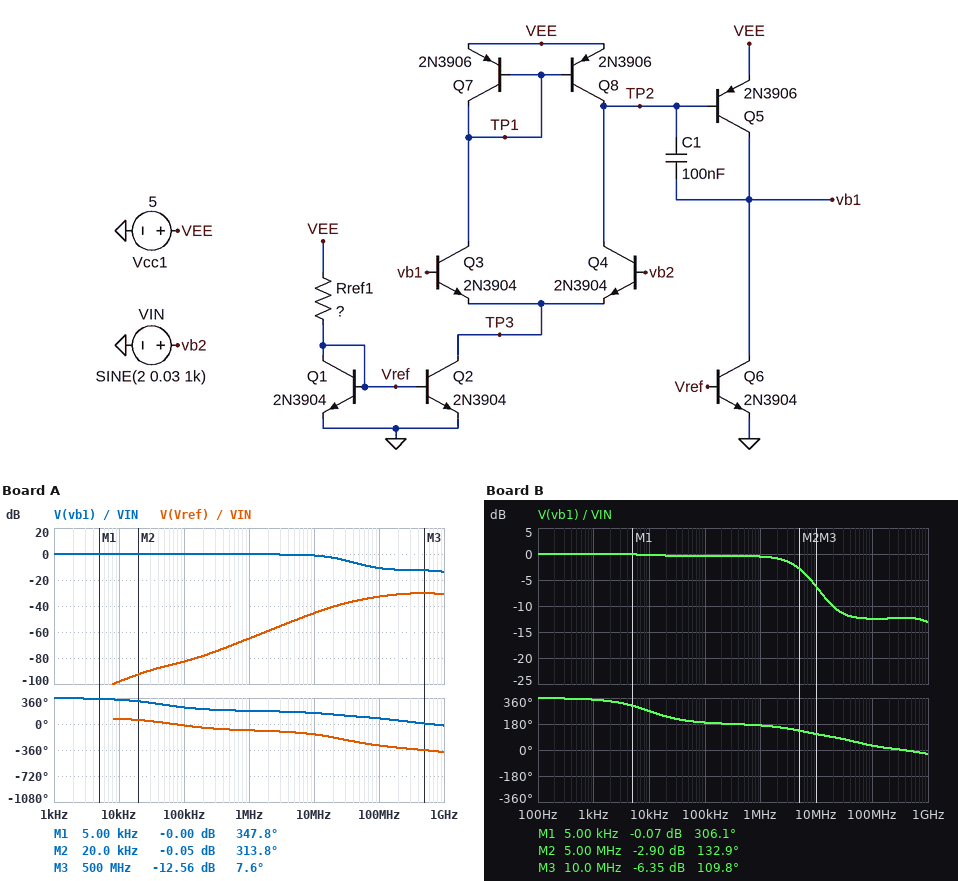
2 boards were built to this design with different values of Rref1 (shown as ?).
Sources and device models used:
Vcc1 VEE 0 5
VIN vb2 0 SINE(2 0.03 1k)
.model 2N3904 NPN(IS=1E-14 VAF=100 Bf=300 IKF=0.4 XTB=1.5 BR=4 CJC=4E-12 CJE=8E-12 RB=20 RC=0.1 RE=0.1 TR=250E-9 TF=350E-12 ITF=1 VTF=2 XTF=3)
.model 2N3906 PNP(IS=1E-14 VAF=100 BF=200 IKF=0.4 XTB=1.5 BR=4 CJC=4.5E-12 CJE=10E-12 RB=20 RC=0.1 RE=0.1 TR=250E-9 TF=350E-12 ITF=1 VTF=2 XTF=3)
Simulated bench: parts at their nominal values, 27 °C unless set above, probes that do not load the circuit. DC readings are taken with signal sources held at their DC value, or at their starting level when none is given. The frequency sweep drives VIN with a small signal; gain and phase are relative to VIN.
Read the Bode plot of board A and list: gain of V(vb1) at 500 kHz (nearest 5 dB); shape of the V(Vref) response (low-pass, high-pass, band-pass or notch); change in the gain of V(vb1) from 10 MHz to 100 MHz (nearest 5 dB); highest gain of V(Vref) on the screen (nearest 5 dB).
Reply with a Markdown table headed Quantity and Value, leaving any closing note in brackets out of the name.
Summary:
| Quantity | Value |
|---|---|
| gain of V(vb1) at 500 kHz | 0 dB |
| shape of the V(Vref) response | high-pass |
| change in the gain of V(vb1) from 10 MHz to 100 MHz | -10 dB |
| highest gain of V(Vref) on the screen | -30 dB |
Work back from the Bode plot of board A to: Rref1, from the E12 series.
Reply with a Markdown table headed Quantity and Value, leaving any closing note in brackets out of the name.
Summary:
| Quantity | Value |
|---|---|
| Rref1, from the E12 series | 5.6 kΩ |
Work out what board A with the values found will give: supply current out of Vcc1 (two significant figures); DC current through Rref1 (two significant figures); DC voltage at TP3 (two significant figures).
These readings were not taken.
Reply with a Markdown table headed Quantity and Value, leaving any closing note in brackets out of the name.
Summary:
| Quantity | Value |
|---|---|
| supply current out of Vcc1 | 2.3 mA |
| DC current through Rref1 | 780 µA |
| DC voltage at TP3 | 1.4 V |
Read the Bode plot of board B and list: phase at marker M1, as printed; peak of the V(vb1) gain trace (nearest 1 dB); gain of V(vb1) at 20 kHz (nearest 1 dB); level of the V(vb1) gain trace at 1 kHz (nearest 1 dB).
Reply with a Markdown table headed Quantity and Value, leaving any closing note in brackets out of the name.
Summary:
| Quantity | Value |
|---|---|
| phase at marker M1, as printed | 306.1 deg |
| peak of the V(vb1) gain trace | 0 dB |
| gain of V(vb1) at 20 kHz | 0 dB |
| level of the V(vb1) gain trace at 1 kHz | 0 dB |
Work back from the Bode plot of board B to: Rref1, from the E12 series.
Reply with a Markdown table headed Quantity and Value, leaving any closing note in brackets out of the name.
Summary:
| Quantity | Value |
|---|---|
| Rref1, from the E12 series | 27 kΩ |
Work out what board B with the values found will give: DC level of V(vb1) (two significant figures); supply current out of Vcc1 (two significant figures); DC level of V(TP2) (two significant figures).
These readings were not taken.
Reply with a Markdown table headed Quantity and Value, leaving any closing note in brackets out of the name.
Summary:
| Quantity | Value |
|---|---|
| DC level of V(vb1) | 2.0 V |
| supply current out of Vcc1 | 490 µA |
| DC level of V(TP2) | 4.4 V |
